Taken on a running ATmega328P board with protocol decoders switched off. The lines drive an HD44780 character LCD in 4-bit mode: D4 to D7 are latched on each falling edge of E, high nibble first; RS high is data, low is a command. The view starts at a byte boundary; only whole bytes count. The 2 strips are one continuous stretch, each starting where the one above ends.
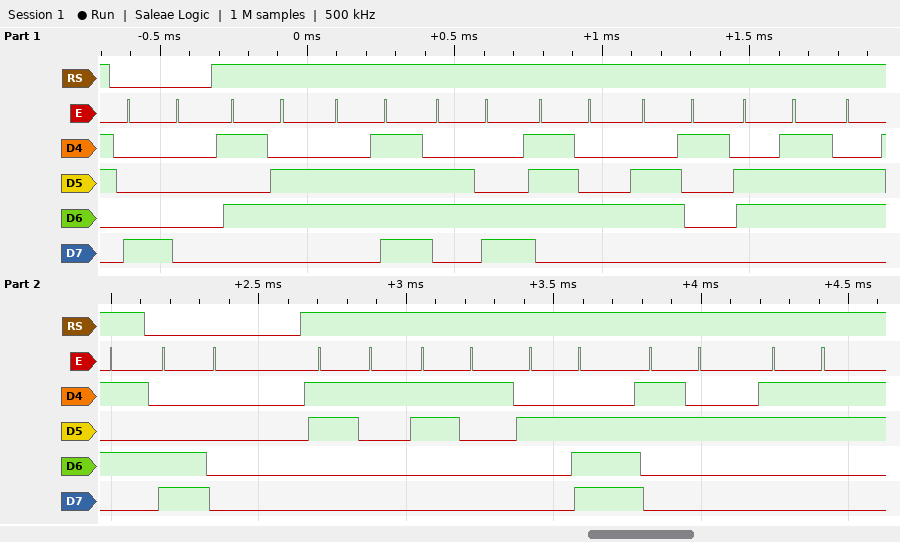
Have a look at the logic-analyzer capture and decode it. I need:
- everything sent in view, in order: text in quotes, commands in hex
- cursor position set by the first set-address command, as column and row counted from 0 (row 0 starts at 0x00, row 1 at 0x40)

0x80 "Voltage" 0xC0 "11.23"
column 0, row 0
